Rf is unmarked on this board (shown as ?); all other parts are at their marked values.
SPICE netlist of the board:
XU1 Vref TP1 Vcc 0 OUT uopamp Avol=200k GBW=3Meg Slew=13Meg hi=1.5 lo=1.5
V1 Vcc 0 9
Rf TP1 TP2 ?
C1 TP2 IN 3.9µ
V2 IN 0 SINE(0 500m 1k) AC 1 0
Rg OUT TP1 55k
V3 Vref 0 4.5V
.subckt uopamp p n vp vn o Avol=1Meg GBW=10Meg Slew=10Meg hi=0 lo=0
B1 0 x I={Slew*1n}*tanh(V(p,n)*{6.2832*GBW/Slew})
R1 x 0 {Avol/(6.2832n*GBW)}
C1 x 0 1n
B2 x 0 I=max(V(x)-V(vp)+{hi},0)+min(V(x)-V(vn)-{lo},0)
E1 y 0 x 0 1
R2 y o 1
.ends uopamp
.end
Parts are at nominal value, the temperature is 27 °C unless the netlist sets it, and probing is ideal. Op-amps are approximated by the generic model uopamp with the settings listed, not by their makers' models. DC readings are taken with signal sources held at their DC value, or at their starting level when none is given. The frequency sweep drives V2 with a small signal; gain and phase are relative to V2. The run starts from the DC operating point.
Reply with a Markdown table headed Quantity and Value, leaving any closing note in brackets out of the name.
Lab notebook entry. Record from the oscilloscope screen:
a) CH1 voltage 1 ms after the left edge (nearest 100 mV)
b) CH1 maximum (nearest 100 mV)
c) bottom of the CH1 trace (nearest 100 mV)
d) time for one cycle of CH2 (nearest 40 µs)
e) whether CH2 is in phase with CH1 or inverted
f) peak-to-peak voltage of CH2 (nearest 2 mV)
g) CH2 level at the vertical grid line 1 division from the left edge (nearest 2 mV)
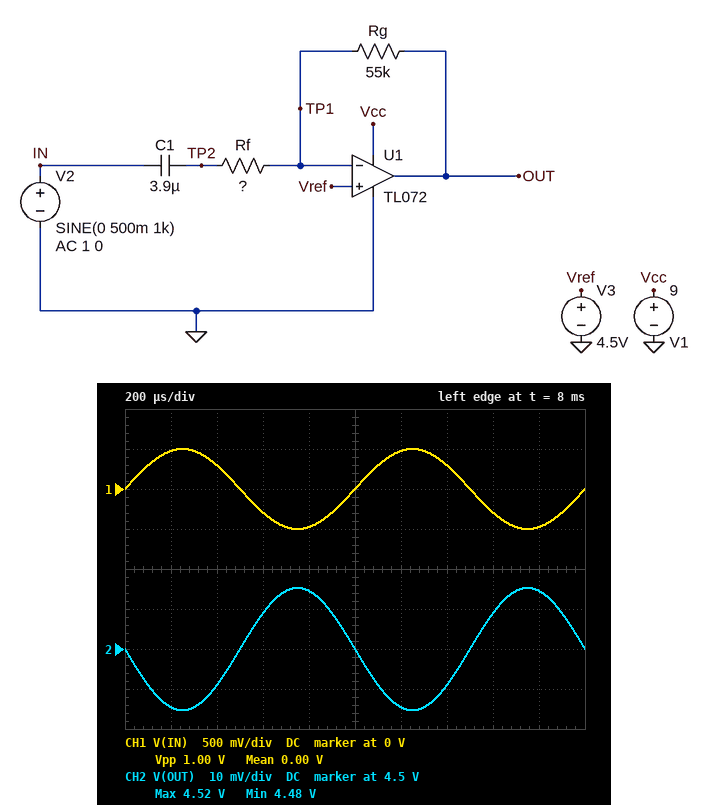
| Quantity | Value |
|---|---|
| CH1 voltage 1 ms after the left edge | 0 V |
| CH1 maximum | 500 mV |
| bottom of the CH1 trace | -500 mV |
| time for one cycle of CH2 | 1.00 ms |
| whether CH2 is in phase with CH1 or inverted | inverted |
| peak-to-peak voltage of CH2 | 30 mV |
| CH2 level at the vertical grid line 1 division from the left edge | 4.486 V |
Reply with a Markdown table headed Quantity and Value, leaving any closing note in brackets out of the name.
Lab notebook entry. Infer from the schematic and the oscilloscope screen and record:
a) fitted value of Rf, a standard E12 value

| Quantity | Value |
|---|---|
| fitted value of Rf, a standard E12 value | 1.8 MΩ |
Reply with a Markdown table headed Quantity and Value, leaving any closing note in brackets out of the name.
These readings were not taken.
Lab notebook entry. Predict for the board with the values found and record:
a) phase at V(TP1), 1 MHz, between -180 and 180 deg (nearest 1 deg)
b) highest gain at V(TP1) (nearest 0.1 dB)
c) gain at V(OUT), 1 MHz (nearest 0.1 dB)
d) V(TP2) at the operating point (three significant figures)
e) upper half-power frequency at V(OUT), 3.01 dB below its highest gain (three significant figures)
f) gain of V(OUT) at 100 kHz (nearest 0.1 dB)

| Quantity | Value |
|---|---|
| phase at V(TP1), 1 MHz, between -180 and 180 deg | 71 deg |
| highest gain at V(TP1) | -30.6 dB |
| gain at V(OUT), 1 MHz | -30.8 dB |
| V(TP2) at the operating point | 4.50 V |
| upper half-power frequency at V(OUT), 3.01 dB below its highest gain | 2.91 MHz |
| gain of V(OUT) at 100 kHz | -30.3 dB |
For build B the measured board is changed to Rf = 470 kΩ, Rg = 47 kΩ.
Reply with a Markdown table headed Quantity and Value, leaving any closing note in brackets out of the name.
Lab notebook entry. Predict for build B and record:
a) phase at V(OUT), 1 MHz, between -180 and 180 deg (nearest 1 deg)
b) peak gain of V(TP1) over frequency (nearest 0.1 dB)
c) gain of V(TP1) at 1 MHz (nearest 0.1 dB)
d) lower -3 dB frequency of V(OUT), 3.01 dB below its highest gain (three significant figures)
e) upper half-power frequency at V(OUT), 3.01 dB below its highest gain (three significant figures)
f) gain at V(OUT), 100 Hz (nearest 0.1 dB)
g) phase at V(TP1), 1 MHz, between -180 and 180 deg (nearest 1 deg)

| Quantity | Value |
|---|---|
| phase at V(OUT), 1 MHz, between -180 and 180 deg | 160 deg |
| peak gain of V(TP1) over frequency | -20.8 dB |
| gain of V(TP1) at 1 MHz | -30.1 dB |
| lower -3 dB frequency of V(OUT), 3.01 dB below its highest gain | 86.8 mHz |
| upper half-power frequency at V(OUT), 3.01 dB below its highest gain | 2.73 MHz |
| gain at V(OUT), 100 Hz | -20.0 dB |
| phase at V(TP1), 1 MHz, between -180 and 180 deg | 70 deg |
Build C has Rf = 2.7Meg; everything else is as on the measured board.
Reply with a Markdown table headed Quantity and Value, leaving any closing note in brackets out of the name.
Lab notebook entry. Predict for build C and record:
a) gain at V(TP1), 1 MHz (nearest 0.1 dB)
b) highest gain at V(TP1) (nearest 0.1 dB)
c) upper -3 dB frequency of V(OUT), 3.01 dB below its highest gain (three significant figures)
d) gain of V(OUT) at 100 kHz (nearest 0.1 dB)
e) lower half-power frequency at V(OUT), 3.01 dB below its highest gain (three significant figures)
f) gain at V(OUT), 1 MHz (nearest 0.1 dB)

| Quantity | Value |
|---|---|
| gain at V(TP1), 1 MHz | -43.8 dB |
| highest gain at V(TP1) | -34.0 dB |
| upper -3 dB frequency of V(OUT), 3.01 dB below its highest gain | 2.94 MHz |
| gain of V(OUT) at 100 kHz | -33.8 dB |
| lower half-power frequency at V(OUT), 3.01 dB below its highest gain | 15.1 mHz |
| gain at V(OUT), 1 MHz | -34.3 dB |
